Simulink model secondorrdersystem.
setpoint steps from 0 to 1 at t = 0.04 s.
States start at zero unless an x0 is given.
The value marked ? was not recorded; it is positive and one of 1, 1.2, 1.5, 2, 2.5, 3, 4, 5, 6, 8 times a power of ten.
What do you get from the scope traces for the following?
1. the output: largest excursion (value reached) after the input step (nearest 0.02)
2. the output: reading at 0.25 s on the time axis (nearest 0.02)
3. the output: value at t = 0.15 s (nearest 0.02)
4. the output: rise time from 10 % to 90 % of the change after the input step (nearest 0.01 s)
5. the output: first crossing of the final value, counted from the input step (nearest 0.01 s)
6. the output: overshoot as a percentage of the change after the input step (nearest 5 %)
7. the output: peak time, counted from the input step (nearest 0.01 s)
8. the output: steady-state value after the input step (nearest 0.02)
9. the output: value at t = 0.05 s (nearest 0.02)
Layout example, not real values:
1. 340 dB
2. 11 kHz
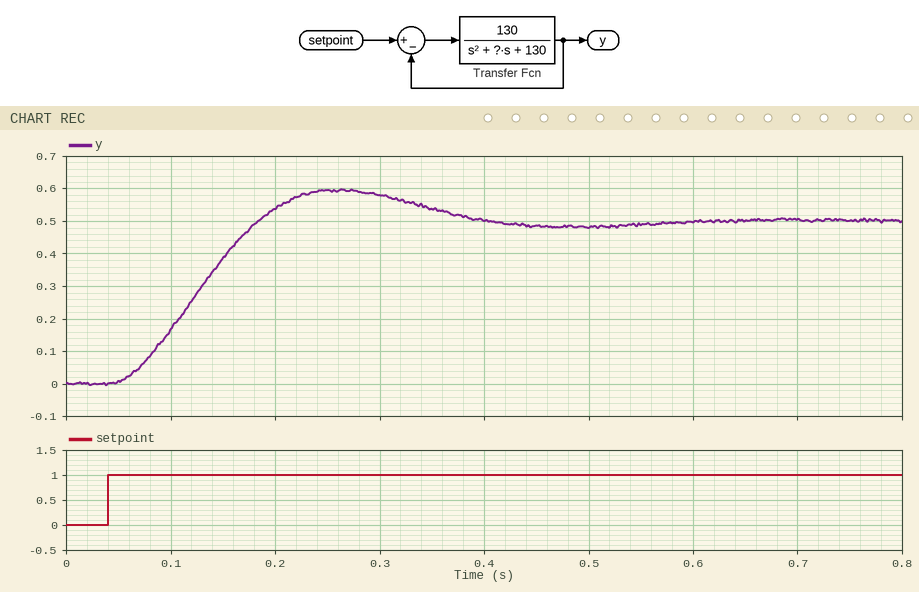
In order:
1. 0.60
2. 0.60
3. 0.38
4. 0.10 s
5. 0.14 s
6. 20 %
7. 0.22 s
8. 0.50
9. 0.00
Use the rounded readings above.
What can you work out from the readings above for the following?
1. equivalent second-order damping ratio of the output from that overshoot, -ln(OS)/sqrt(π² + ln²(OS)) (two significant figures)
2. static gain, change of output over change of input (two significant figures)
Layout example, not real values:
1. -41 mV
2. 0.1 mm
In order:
1. 0.46
2. 0.50
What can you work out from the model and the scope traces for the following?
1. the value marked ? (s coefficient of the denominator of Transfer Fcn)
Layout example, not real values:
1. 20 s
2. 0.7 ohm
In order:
1. 15
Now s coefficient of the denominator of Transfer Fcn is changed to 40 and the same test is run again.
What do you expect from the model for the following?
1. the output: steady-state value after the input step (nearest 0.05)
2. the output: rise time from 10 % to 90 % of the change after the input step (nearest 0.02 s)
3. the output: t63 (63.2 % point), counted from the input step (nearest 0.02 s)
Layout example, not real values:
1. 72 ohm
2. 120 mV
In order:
1. 0.50
2. 0.28 s
3. 0.16 s
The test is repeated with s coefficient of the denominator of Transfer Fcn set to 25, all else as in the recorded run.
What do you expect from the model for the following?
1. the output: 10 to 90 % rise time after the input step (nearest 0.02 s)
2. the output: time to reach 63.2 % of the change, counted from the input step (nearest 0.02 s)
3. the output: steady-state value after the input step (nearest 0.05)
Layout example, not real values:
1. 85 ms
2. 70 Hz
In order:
1. 0.14 s
2. 0.12 s
3. 0.50
